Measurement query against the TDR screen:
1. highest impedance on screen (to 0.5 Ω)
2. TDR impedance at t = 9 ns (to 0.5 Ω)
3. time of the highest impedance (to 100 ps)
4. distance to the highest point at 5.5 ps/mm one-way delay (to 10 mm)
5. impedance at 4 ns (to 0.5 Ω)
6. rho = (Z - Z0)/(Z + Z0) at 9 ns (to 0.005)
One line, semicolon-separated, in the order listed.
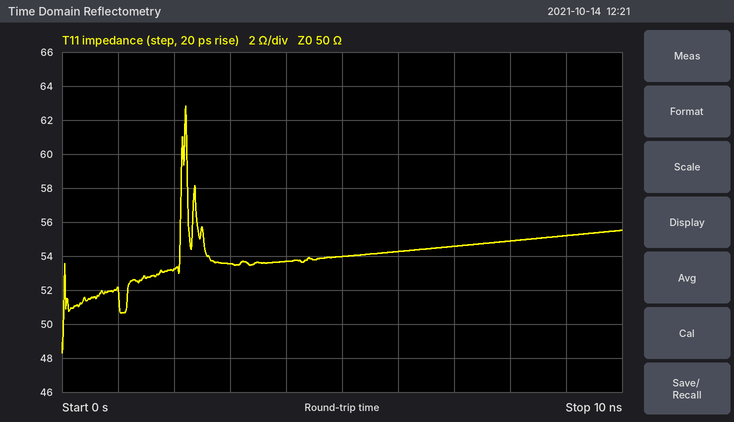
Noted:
63.0 Ω; 55.0 Ω; 2.2 ns; 200 mm; 53.5 Ω; +0.050
